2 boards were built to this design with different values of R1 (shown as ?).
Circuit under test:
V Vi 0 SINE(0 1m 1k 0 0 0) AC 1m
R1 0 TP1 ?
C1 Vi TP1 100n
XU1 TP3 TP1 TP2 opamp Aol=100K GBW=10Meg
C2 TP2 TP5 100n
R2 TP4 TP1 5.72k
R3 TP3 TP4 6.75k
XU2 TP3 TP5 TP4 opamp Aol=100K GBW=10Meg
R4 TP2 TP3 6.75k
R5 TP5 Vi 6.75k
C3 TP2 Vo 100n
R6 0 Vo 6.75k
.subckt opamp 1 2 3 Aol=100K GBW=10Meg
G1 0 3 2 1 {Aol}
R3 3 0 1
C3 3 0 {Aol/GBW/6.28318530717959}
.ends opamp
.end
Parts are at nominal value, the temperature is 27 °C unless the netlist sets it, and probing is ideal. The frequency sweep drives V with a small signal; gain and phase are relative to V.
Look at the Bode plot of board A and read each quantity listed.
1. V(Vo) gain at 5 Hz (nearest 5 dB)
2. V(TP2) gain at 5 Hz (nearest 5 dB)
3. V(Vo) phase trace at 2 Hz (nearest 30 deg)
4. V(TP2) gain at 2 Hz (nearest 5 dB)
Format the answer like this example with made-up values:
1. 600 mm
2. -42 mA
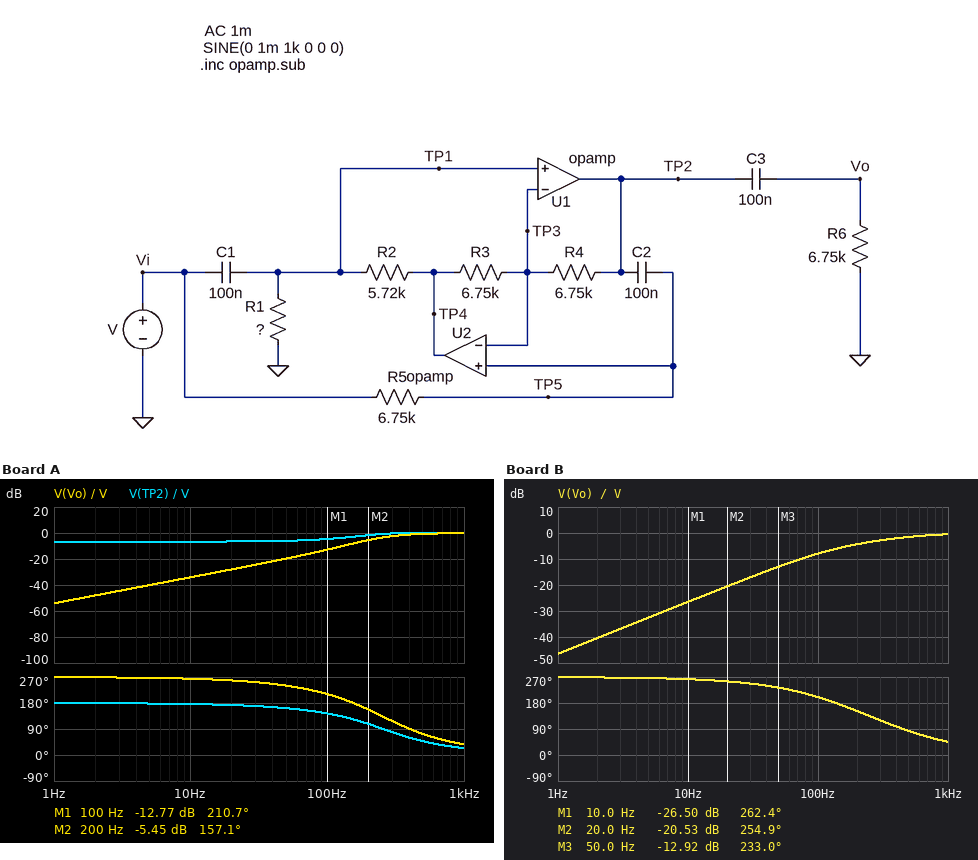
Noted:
1. -40 dB
2. -5 dB
3. 270 deg
4. -5 dB
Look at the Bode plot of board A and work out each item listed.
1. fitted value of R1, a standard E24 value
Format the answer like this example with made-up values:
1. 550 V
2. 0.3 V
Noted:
1. 3.9 kΩ
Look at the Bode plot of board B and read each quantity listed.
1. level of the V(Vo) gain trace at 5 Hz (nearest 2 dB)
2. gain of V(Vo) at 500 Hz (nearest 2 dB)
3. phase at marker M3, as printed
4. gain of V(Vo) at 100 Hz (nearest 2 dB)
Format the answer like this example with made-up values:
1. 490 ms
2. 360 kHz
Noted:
1. -32 dB
2. -2 dB
3. 233.0 deg
4. -8 dB
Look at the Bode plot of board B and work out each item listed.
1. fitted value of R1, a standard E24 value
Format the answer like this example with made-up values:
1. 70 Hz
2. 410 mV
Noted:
1. 2.7 kΩ
